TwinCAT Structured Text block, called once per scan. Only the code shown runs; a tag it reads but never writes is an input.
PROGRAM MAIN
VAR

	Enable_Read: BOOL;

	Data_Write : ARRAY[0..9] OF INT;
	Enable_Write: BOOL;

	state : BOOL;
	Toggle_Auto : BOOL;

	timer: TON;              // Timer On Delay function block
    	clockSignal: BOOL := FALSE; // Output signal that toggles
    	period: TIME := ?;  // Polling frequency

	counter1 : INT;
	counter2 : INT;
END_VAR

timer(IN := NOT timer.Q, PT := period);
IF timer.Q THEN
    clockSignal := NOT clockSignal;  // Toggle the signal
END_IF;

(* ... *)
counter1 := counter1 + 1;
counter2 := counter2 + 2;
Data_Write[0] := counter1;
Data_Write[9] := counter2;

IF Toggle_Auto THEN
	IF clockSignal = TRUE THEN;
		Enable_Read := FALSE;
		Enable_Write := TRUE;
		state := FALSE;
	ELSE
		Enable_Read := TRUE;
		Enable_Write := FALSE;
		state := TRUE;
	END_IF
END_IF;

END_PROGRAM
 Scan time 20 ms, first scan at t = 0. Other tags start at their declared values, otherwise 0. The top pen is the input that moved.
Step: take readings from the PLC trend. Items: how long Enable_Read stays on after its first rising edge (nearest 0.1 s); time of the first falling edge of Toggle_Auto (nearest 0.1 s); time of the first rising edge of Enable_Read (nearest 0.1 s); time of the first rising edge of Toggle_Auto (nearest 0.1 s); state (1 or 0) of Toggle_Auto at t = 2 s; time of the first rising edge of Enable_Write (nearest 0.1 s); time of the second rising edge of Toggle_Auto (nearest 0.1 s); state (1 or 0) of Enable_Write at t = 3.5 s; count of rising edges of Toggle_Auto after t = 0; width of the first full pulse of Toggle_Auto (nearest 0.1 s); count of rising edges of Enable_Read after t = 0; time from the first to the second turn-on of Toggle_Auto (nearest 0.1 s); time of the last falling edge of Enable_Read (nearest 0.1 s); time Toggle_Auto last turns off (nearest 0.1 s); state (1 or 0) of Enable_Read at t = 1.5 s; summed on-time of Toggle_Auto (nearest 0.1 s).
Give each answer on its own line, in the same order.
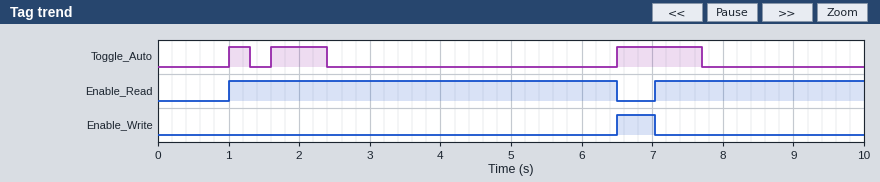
5.5 s
1.3 s
1.0 s
1.0 s
1
6.5 s
1.6 s
0
3
0.3 s
2
0.6 s
6.5 s
7.7 s
1
2.3 s
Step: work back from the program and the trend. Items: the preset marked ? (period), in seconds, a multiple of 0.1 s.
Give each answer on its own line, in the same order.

3.5 s
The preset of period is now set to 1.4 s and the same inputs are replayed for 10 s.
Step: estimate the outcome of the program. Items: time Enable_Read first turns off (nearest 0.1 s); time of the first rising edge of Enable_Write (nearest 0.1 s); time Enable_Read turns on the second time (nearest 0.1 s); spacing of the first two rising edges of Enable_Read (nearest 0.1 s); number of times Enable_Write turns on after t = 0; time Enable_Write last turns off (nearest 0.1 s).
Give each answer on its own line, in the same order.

1.6 s
1.6 s
6.5 s
5.5 s
2
6.5 s
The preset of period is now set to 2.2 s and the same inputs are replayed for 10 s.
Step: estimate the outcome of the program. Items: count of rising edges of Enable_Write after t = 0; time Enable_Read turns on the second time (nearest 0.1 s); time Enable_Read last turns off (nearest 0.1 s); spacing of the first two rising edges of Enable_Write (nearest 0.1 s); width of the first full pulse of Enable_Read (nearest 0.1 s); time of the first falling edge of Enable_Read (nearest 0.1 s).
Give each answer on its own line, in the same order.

2
6.5 s
6.7 s
4.5 s
1.2 s
2.2 s
